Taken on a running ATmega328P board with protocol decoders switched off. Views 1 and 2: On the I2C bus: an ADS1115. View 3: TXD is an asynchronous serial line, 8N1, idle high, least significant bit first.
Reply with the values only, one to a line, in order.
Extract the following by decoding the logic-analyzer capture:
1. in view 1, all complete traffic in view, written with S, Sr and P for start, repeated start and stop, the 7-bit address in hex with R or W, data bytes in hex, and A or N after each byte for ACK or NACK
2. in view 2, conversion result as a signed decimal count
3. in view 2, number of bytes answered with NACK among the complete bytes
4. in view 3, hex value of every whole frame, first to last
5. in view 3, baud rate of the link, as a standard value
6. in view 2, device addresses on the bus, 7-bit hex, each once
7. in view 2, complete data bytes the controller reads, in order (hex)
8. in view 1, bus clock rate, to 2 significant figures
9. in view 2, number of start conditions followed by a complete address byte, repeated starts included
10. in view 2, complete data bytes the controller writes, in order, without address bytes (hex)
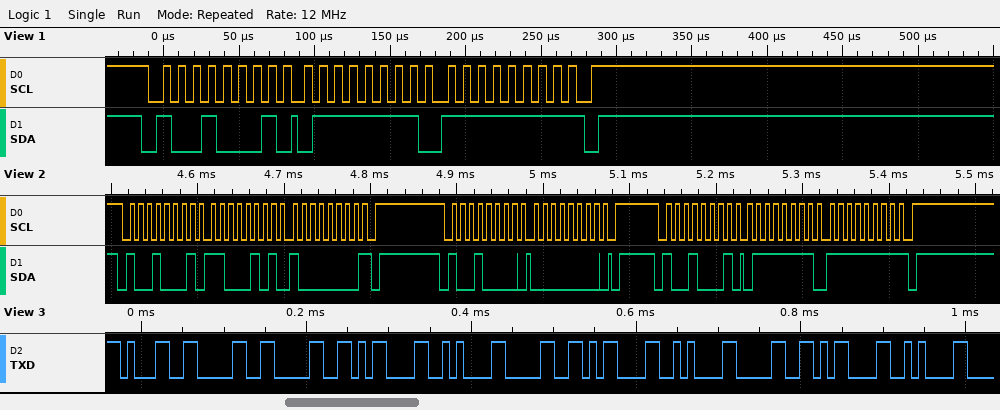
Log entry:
S 48R A 7F A FF N P
32767
2
0x31 0x30 0x30 0x0D 0x0A 0x30 0x0D 0x0A 0x30 0x0D 0x0A
115200 baud
0x48
C5 80 7F FF
100 kHz
3
00
